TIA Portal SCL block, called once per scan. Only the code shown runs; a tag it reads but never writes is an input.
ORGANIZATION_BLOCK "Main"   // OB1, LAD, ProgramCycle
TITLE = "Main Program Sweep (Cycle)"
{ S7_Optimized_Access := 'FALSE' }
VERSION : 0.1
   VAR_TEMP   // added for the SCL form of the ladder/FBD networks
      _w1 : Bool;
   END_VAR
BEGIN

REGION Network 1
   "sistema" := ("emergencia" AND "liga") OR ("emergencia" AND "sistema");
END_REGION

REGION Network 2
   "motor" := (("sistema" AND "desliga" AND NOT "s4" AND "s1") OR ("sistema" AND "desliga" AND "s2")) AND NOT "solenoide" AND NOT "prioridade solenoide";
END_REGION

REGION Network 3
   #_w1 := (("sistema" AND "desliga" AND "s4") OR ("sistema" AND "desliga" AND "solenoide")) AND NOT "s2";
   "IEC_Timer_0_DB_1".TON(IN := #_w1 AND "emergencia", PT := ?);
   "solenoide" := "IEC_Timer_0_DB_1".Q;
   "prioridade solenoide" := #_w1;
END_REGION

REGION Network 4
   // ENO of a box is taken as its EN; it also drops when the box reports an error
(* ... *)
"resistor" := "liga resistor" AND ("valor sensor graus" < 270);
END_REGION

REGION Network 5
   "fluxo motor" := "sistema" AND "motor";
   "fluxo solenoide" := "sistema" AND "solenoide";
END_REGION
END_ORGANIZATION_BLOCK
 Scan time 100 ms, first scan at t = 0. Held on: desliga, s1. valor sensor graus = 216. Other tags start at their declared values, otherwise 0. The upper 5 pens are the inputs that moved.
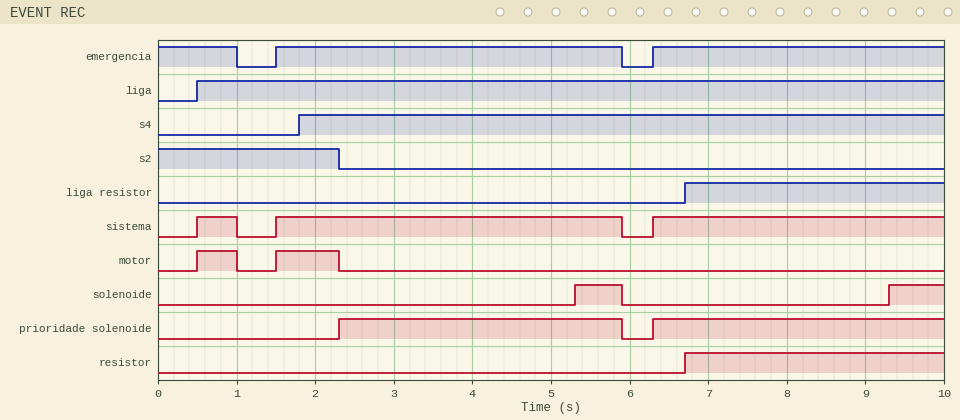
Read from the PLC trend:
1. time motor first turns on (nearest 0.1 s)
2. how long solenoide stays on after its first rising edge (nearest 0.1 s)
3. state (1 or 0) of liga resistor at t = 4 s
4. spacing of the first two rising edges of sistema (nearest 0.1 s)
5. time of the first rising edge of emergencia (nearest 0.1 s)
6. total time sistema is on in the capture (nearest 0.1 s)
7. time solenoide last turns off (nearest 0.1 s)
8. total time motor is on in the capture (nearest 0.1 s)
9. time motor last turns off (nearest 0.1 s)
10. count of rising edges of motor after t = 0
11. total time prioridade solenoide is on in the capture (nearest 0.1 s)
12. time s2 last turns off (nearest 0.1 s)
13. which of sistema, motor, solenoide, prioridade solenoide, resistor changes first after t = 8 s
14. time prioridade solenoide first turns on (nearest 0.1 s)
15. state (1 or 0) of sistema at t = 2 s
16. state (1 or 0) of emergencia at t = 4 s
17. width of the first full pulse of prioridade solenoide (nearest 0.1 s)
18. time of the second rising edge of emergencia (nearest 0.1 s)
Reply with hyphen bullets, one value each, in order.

- 0.5 s
- 0.6 s
- 0
- 1.0 s
- 1.5 s
- 8.6 s
- 5.9 s
- 1.3 s
- 2.3 s
- 2
- 7.3 s
- 2.3 s
- solenoide
- 2.3 s
- 1
- 1
- 3.6 s
- 6.3 s
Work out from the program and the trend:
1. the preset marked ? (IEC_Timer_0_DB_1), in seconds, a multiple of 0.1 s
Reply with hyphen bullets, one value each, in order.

- 3.0 s
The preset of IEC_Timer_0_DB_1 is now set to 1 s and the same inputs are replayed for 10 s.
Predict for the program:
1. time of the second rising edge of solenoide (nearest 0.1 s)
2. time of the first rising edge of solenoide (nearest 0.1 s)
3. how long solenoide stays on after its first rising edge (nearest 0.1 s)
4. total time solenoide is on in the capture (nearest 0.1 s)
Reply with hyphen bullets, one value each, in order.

- 7.3 s
- 3.3 s
- 2.6 s
- 5.3 s
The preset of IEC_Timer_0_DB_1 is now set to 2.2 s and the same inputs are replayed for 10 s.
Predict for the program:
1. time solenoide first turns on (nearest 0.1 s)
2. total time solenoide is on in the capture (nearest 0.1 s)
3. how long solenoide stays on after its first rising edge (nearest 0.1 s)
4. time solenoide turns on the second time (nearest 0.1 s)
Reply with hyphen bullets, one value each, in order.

- 4.5 s
- 2.9 s
- 1.4 s
- 8.5 s
